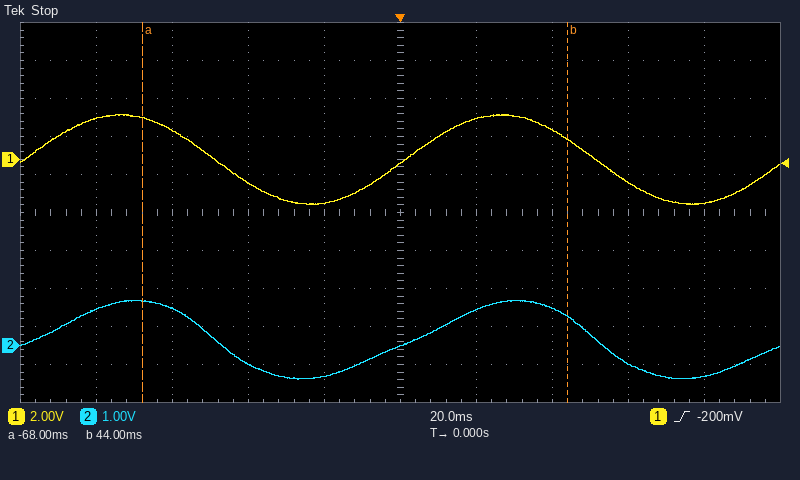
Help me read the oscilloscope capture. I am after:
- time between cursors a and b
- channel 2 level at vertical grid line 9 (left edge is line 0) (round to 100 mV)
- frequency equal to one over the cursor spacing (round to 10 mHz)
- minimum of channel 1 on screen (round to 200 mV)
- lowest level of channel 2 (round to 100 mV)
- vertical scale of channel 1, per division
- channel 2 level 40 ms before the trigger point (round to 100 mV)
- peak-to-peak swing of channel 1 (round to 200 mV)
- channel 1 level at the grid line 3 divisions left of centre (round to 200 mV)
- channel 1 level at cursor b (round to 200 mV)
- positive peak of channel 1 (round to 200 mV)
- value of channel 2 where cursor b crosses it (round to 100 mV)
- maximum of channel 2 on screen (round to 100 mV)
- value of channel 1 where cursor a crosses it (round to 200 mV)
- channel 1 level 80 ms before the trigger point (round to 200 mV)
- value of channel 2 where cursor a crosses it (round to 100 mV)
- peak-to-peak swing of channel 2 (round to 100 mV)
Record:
112 ms
-800 mV
8.93 Hz
-2.4 V
-900 mV
2 V
-500 mV
4.8 V
1.6 V
1.0 V
2.4 V
800 mV
1.2 V
2.2 V
2.2 V
1.2 V
2.1 V
